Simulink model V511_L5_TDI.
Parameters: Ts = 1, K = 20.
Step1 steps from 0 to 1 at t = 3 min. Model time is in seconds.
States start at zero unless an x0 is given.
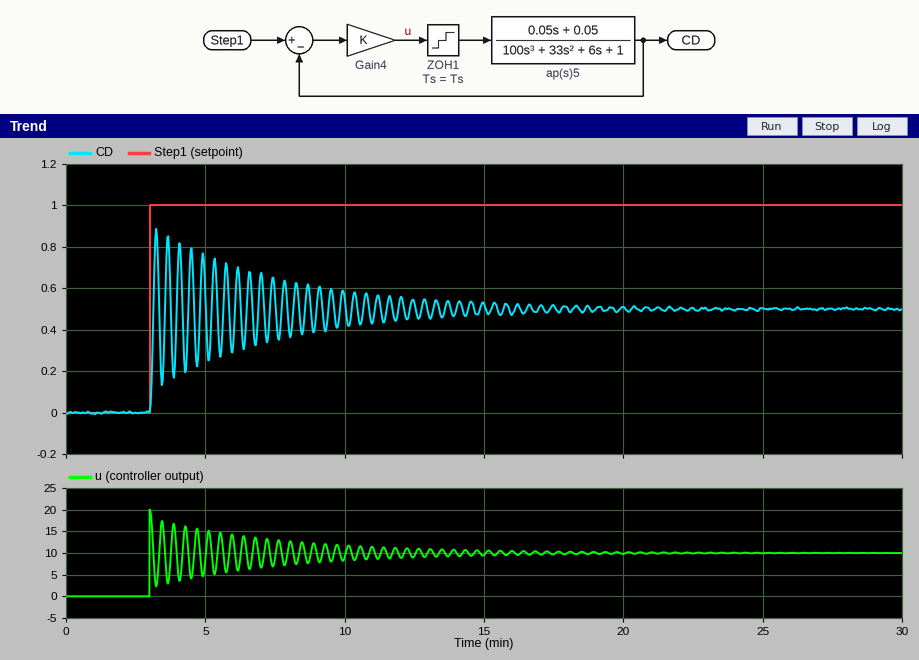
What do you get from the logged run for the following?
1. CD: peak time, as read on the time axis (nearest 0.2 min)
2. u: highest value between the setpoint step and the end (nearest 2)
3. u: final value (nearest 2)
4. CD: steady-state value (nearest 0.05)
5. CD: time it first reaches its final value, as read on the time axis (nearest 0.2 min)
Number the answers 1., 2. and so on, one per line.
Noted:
1. 3.2 min
2. 20
3. 10
4. 0.50
5. 3.2 min
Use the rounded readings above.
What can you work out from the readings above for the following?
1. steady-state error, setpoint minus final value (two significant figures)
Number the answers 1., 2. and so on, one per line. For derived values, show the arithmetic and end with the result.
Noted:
1. 1 - 0.5 = 0.50
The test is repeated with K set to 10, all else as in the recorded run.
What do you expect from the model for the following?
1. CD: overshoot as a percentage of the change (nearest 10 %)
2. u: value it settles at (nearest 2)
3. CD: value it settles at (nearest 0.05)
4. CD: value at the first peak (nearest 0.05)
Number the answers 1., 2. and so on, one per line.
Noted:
1. 60 %
2. 6
3. 0.35
4. 0.55
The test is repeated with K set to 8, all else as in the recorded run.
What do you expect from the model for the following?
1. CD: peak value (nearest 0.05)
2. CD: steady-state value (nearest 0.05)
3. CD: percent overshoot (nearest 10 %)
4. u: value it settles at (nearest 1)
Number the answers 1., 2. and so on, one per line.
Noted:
1. 0.45
2. 0.30
3. 60 %
4. 6
